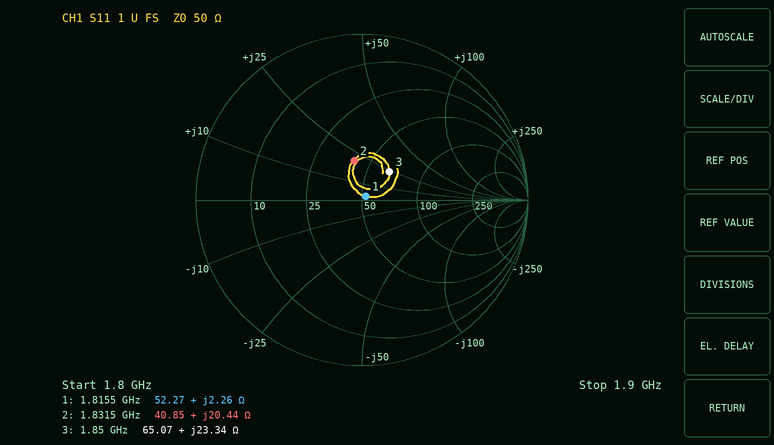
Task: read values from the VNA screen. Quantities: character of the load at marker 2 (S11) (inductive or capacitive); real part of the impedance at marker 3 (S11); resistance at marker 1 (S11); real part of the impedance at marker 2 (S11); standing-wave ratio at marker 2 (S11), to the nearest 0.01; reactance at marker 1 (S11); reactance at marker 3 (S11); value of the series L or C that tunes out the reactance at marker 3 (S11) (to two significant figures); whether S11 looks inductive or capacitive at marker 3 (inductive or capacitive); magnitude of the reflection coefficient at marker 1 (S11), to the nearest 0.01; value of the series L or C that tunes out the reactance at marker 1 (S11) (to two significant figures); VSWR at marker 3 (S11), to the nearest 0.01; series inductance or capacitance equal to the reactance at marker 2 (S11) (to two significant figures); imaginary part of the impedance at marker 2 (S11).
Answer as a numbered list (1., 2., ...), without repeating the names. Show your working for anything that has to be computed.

1. inductive
2. 65.07 Ω
3. 52.27 Ω
4. 40.85 Ω
5. 1.63
6. +2.26 Ω
7. +23.34 Ω
8. C = 1/(2π × 1.85 GHz × 23.34 Ω) ≈ 3.7 pF
9. inductive
10. 0.03
11. C = 1/(2π × 1.8155 GHz × 2.26 Ω) ≈ 39 pF
12. 1.62
13. L = 20.44 Ω/(2π × 1.8315 GHz) ≈ 1.8 nH
14. +20.44 Ω
